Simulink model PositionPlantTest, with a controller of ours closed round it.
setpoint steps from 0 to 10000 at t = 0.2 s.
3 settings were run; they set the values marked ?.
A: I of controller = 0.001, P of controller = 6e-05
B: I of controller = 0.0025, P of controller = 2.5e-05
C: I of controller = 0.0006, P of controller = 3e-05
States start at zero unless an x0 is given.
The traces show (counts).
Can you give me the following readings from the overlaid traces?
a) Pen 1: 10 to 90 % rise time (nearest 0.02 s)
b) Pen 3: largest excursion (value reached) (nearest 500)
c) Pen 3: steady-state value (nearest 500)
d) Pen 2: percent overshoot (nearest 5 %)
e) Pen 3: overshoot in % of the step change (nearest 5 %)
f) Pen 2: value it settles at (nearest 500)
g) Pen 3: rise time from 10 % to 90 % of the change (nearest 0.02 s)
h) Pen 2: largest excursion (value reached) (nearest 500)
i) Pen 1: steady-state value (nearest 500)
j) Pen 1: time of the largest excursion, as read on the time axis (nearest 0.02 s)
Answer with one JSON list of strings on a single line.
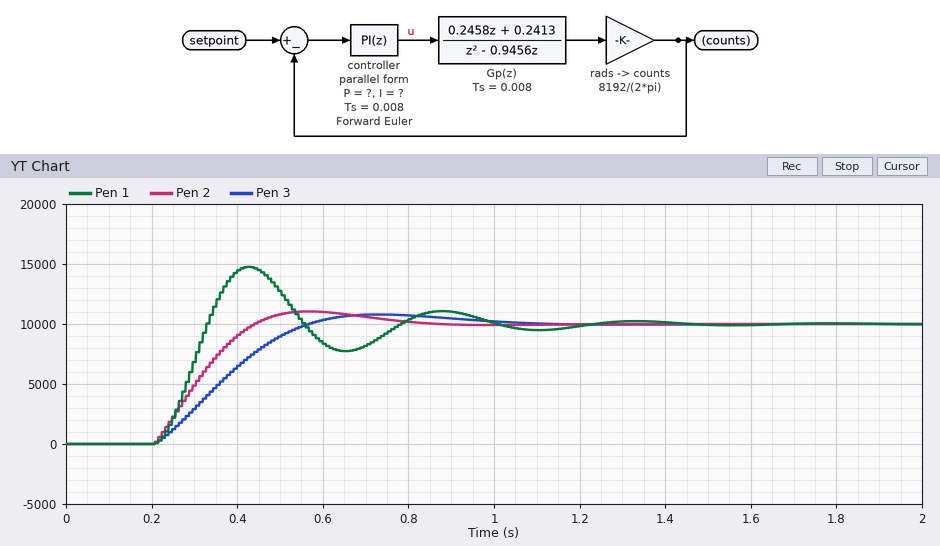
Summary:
["0.08 s", "11000", "10000", "10 %", "10 %", "10000", "0.26 s", "11000", "10000", "0.42 s"]
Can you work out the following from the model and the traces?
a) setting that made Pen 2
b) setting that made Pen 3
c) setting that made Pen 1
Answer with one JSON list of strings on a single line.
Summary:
["A", "C", "B"]
